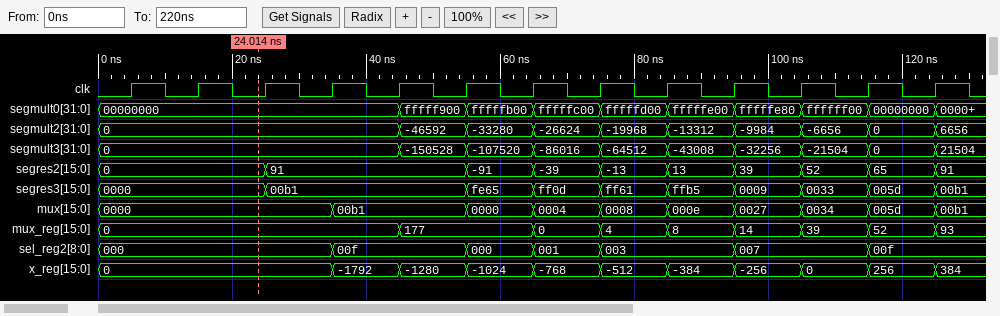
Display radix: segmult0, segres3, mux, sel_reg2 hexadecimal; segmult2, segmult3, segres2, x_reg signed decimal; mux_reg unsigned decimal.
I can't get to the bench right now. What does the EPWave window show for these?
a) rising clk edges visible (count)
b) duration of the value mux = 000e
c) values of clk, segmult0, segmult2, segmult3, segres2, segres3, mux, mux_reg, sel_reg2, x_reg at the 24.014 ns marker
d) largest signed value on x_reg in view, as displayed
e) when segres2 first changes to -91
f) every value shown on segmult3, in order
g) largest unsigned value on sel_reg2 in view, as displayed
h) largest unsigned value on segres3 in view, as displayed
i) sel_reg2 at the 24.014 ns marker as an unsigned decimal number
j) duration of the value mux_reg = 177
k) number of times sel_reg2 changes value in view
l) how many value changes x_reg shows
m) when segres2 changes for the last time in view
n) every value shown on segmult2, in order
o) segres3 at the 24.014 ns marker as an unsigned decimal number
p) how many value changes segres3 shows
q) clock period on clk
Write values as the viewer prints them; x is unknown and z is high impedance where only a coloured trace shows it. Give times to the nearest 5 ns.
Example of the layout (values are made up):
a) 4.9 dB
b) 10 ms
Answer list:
a) 13
b) 10 ns
c) clk=0, segmult0=00000000, segmult2=0, segmult3=0, segres2=0, segres3=0000, mux=0000, mux_reg=0, sel_reg2=000, x_reg=0
d) 384
e) 55 ns
f) 0, -150528, -107520, -86016, -64512, -43008, -32256, -21504, 0, 21504
g) 00f
h) ffb5
i) 0
j) 20 ns
k) 6
l) 10
m) 125 ns
n) 0, -46592, -33280, -26624, -19968, -13312, -9984, -6656, 0, 6656
o) 0
p) 9
q) 10 ns
